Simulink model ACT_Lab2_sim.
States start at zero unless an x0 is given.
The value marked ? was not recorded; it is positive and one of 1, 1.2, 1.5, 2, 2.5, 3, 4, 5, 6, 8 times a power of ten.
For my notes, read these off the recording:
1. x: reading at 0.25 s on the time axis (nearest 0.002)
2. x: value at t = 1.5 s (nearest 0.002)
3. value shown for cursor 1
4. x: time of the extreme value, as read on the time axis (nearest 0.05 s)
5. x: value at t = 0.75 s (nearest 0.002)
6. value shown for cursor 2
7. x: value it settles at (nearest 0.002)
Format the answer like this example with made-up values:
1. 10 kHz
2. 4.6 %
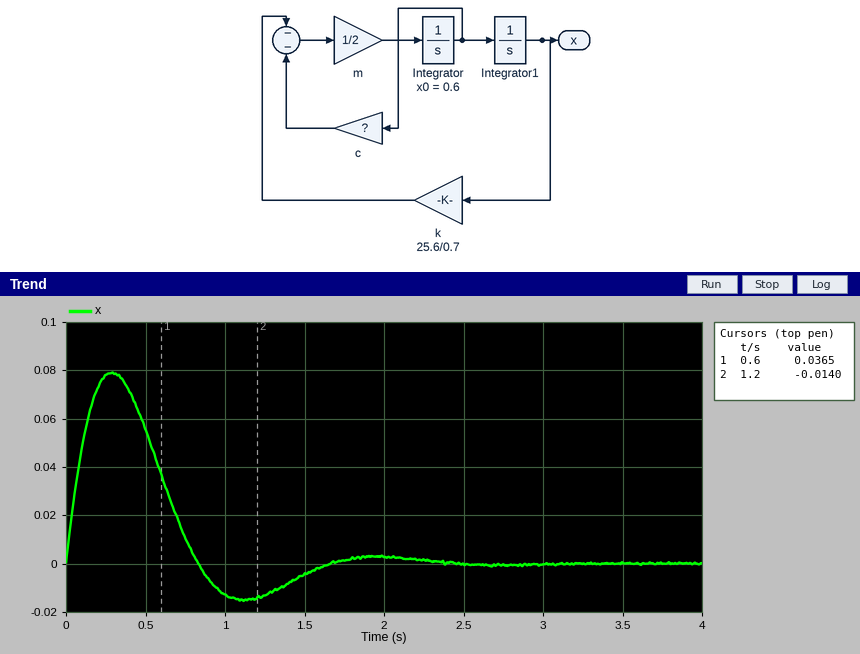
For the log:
1. 0.078
2. -0.004
3. 0.0365
4. 0.30 s
5. 0.010
6. -0.0140
7. 0.000
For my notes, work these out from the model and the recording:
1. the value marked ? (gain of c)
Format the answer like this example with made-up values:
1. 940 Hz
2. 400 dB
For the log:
1. 8
